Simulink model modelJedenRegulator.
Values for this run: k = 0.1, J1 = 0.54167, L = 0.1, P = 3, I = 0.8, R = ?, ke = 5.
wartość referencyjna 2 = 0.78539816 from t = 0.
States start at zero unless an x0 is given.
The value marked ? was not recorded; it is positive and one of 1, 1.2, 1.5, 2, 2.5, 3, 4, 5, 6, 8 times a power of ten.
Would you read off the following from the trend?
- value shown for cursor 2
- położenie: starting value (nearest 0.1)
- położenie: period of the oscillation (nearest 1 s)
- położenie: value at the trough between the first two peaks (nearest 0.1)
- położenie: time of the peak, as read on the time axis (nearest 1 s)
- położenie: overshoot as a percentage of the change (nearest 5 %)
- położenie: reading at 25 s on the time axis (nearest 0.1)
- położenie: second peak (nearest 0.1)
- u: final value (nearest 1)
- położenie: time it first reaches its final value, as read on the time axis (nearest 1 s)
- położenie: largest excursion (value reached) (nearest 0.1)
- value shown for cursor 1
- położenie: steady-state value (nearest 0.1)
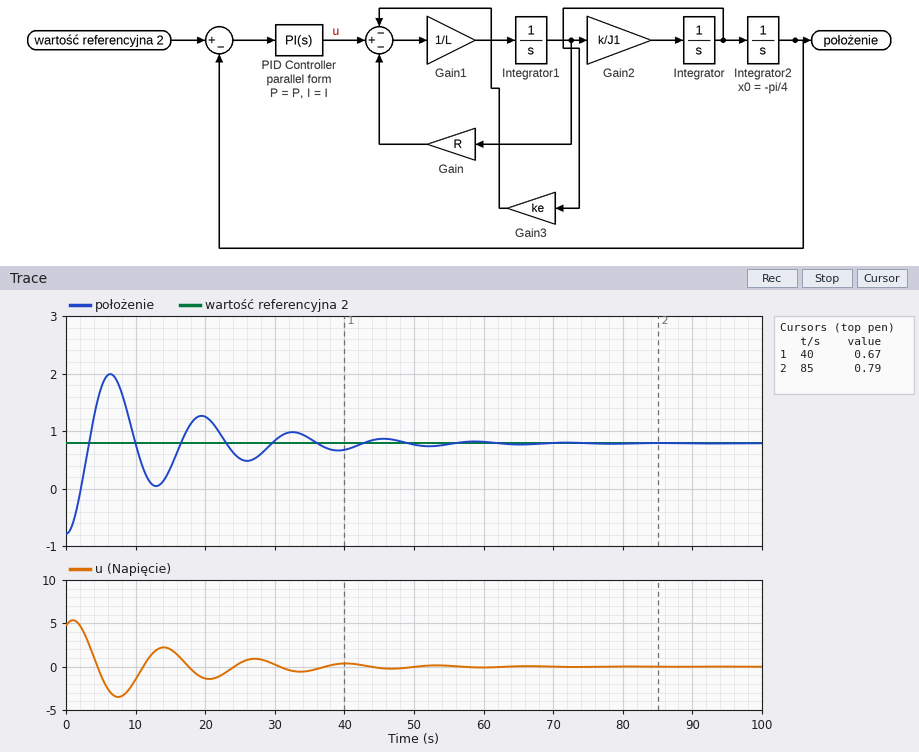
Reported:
0.79
-0.8
13 s
0.0
6 s
75 %
0.5
1.3
0
3 s
2.0
0.67
0.8
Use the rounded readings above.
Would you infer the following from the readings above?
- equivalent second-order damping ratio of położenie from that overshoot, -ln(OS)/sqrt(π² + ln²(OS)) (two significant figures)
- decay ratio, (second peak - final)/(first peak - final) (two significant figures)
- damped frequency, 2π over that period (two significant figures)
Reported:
0.091
0.42
0.48 rad/s
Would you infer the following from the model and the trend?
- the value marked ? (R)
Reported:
2
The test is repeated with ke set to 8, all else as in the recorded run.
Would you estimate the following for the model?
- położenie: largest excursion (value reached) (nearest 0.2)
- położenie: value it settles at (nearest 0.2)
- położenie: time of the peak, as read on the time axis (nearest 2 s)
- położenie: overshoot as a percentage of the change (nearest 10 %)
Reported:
1.6
0.8
8 s
60 %
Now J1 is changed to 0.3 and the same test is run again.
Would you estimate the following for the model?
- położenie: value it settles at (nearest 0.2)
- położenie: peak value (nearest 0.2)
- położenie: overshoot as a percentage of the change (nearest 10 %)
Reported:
0.8
1.6
50 %
